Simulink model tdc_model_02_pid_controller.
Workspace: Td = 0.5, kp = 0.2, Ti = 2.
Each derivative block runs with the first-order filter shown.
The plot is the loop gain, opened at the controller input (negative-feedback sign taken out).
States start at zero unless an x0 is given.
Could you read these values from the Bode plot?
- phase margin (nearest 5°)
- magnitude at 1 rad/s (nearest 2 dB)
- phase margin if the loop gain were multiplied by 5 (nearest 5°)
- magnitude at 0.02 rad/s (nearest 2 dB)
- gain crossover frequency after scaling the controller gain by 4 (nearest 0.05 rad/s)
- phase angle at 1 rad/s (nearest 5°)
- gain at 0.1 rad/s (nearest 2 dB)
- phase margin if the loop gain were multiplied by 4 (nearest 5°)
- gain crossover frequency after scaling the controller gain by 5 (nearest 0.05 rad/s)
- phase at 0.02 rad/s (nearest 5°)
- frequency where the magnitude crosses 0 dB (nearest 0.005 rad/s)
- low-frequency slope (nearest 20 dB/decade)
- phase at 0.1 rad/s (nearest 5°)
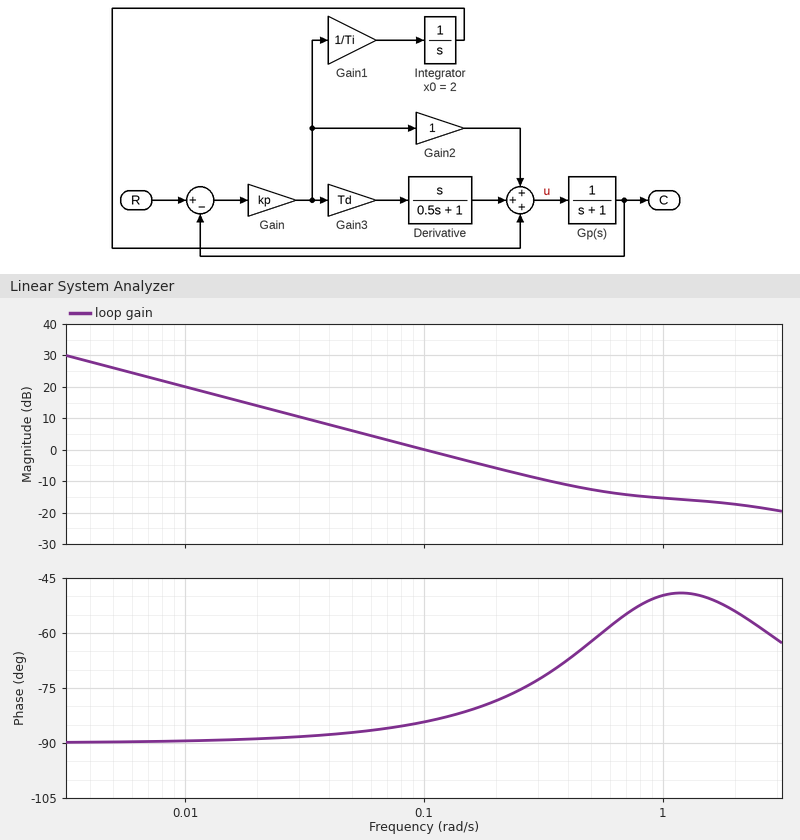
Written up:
95°
-16 dB
125°
14 dB
0.45 rad/s
-50°
0 dB
115°
0.65 rad/s
-90°
0.100 rad/s
-20 dB/decade
-85°
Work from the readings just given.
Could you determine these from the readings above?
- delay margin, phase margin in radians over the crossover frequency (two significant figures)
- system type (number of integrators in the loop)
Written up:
17 s
1
